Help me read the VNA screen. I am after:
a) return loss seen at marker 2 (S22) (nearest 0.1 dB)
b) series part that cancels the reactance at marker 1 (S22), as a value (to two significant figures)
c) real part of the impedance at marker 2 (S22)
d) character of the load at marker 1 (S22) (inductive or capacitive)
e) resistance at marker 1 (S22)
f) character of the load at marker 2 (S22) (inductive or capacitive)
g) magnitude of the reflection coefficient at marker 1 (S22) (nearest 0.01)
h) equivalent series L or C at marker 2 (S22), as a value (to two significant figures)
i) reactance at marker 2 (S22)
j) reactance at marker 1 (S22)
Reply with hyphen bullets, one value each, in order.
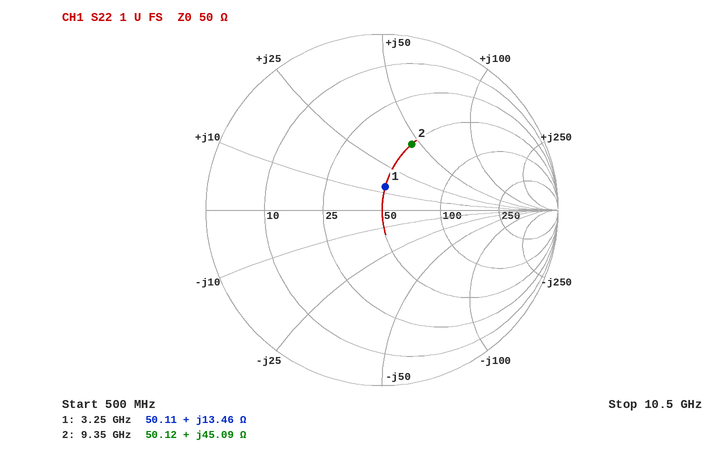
- 7.7 dB
- 3.6 pF
- 50.12 Ω
- inductive
- 50.11 Ω
- inductive
- 0.13
- 770 pH
- +45.09 Ω
- +13.46 Ω
